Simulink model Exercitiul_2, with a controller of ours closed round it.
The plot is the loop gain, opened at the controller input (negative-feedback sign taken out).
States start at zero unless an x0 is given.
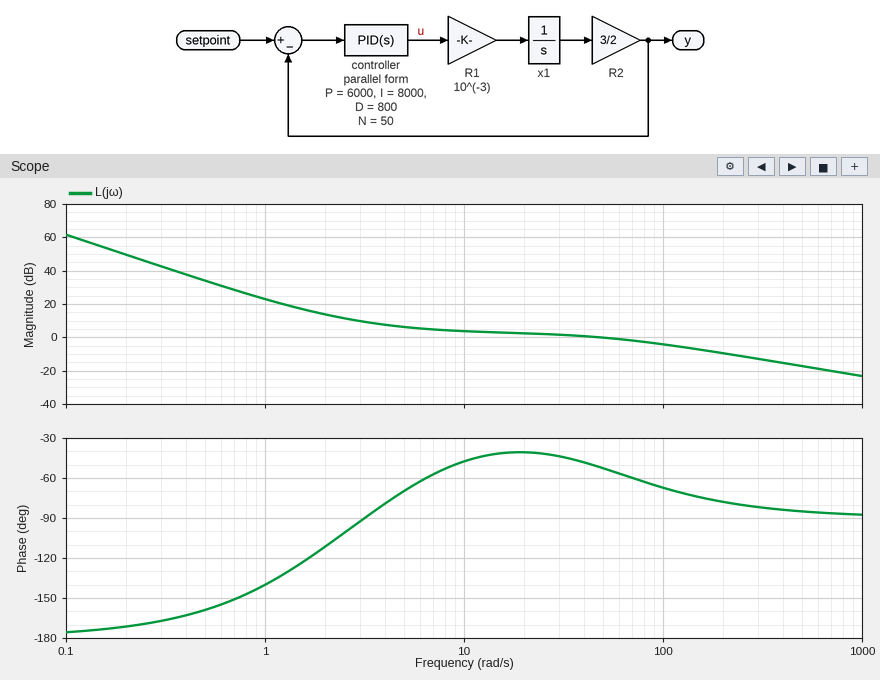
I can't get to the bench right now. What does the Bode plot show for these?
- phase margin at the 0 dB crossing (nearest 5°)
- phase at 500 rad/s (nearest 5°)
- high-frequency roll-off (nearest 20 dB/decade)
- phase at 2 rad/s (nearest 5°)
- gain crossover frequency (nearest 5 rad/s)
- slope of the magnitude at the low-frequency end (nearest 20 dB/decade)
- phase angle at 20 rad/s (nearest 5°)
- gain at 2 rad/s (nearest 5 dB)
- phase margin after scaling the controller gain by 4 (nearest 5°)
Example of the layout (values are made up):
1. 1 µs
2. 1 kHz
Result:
1. 130°
2. -85°
3. -20 dB/decade
4. -110°
5. 50 rad/s
6. -40 dB/decade
7. -40°
8. 15 dB
9. 100°
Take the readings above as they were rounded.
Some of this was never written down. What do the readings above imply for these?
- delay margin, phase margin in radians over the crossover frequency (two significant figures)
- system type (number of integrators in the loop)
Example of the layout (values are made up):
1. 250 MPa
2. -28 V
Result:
1. 0.045 s
2. 2
